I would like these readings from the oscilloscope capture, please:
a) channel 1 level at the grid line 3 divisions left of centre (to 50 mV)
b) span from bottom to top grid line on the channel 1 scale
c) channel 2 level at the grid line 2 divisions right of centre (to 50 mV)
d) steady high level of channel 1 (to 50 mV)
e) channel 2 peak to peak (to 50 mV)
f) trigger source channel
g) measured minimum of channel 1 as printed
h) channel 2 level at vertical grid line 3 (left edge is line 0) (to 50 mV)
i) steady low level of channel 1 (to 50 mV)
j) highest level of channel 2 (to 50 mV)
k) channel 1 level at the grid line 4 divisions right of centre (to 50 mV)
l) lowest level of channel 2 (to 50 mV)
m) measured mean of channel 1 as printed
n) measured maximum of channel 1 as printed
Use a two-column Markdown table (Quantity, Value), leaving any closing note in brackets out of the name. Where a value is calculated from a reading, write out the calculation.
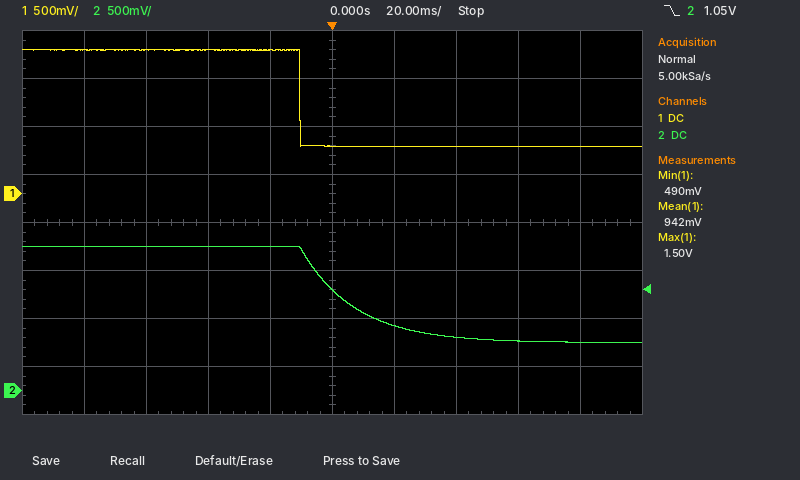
| Quantity | Value |
|---|---|
| channel 1 level at the grid line 3 divisions left of centre | 1.50 V |
| span from bottom to top grid line on the channel 1 scale | 4 V |
| channel 2 level at the grid line 2 divisions right of centre | 550 mV |
| steady high level of channel 1 | 1.50 V |
| channel 2 peak to peak | 1.50 V − (500 mV) = 1.00 V |
| trigger source channel | channel 2 |
| measured minimum of channel 1 as printed | 490 mV |
| channel 2 level at vertical grid line 3 (left edge is line 0) | 1.50 V |
| steady low level of channel 1 | 500 mV |
| highest level of channel 2 | 1.50 V |
| channel 1 level at the grid line 4 divisions right of centre | 500 mV |
| lowest level of channel 2 | 500 mV |
| measured mean of channel 1 as printed | 942 mV |
| measured maximum of channel 1 as printed | 1.50 V |
